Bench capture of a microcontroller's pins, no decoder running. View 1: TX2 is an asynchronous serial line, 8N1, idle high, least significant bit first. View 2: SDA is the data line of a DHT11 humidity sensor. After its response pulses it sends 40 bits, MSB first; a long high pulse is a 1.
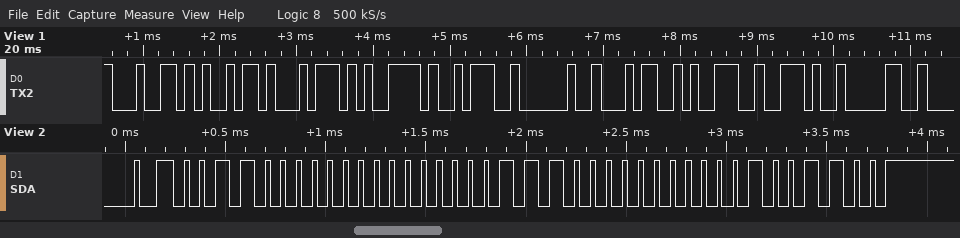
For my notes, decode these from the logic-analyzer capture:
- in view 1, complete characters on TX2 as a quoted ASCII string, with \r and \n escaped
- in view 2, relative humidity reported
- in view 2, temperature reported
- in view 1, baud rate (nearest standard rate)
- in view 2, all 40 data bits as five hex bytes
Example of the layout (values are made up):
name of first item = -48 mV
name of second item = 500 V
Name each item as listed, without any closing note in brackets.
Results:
in view 1, complete characters on TX2 as a quoted ASCII string, with \r and \n escaped = "dity: 49.0"
in view 2, relative humidity reported = 48 %
in view 2, temperature reported = 28.0 °C
in view 1, baud rate = 9600 baud
in view 2, all 40 data bits as five hex bytes = 30 00 1C 00 4C
